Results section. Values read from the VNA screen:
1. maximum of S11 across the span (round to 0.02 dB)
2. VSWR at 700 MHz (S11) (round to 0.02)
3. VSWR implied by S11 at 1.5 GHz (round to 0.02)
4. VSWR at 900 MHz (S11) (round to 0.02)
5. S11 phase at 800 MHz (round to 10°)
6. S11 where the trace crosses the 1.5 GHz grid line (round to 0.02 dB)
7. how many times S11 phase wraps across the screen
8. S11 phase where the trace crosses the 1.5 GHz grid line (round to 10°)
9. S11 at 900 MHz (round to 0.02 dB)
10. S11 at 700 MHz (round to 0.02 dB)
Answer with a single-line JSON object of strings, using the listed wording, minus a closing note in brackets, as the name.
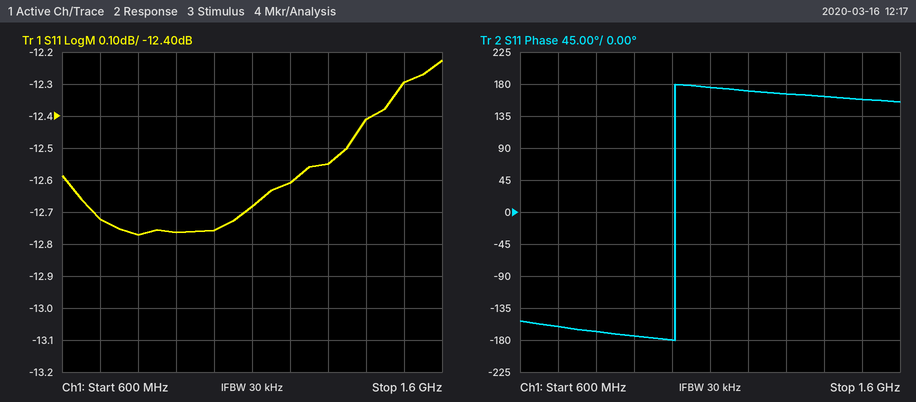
{"maximum of S11 across the span": "-12.22 dB", "VSWR at 700 MHz (S11)": "1.60", "VSWR implied by S11 at 1.5 GHz": "1.64", "VSWR at 900 MHz (S11)": "1.60", "S11 phase at 800 MHz": "-170°", "S11 where the trace crosses the 1.5 GHz grid line": "-12.30 dB", "how many times S11 phase wraps across the screen": "1", "S11 phase where the trace crosses the 1.5 GHz grid line": "160°", "S11 at 900 MHz": "-12.76 dB", "S11 at 700 MHz": "-12.72 dB"}
